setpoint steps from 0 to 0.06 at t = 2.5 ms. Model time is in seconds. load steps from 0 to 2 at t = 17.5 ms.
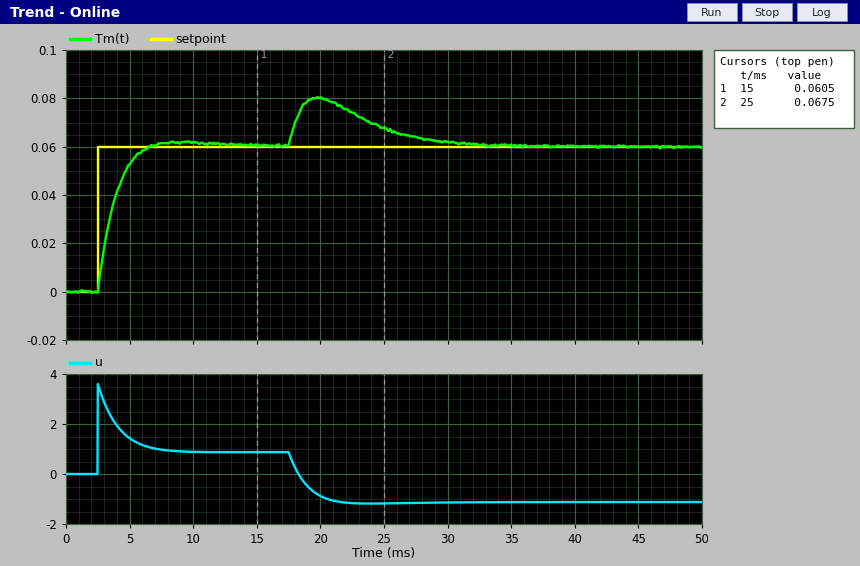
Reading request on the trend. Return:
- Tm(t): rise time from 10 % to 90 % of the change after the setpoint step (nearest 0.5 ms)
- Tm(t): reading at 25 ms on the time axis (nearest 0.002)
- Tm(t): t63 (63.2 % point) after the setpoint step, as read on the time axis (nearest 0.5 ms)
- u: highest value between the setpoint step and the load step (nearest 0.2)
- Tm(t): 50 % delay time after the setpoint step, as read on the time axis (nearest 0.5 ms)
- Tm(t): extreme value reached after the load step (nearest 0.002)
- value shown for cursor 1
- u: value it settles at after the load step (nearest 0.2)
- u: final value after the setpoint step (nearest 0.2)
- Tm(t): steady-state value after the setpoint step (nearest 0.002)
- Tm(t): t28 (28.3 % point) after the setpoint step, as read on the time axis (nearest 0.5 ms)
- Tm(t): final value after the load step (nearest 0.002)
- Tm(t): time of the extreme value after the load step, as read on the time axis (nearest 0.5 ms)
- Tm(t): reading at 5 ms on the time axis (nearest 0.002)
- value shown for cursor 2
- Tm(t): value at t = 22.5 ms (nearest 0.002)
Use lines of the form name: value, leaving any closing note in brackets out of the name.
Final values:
Tm(t): rise time from 10 % to 90 % of the change after the setpoint step: 2.5 ms
Tm(t): reading at 25 ms on the time axis: 0.068
Tm(t): t63 (63.2 % point) after the setpoint step, as read on the time axis: 4.0 ms
u: highest value between the setpoint step and the load step: 3.6
Tm(t): 50 % delay time after the setpoint step, as read on the time axis: 3.5 ms
Tm(t): extreme value reached after the load step: 0.080
value shown for cursor 1: 0.0605
u: value it settles at after the load step: -1.2
u: final value after the setpoint step: 0.8
Tm(t): steady-state value after the setpoint step: 0.060
Tm(t): t28 (28.3 % point) after the setpoint step, as read on the time axis: 3.0 ms
Tm(t): final value after the load step: 0.060
Tm(t): time of the extreme value after the load step, as read on the time axis: 20.0 ms
Tm(t): reading at 5 ms on the time axis: 0.052
value shown for cursor 2: 0.0675
Tm(t): value at t = 22.5 ms: 0.074
